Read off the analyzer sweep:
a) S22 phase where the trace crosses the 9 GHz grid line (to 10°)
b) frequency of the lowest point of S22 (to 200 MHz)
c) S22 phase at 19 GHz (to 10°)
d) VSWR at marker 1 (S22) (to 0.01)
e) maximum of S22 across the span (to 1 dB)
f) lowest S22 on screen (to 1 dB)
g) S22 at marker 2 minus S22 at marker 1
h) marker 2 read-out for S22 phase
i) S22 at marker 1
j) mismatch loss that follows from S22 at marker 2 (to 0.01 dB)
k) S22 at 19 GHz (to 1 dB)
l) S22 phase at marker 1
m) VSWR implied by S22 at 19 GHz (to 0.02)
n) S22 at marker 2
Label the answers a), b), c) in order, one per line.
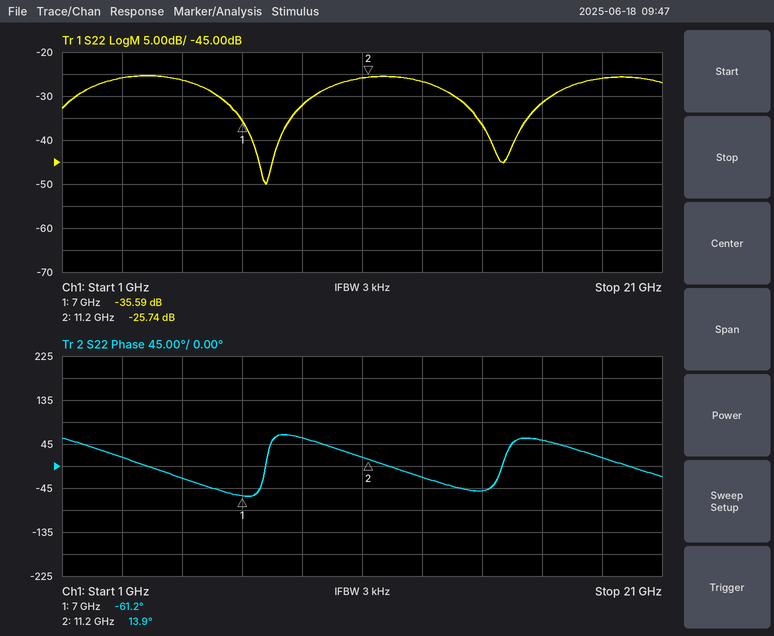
a) 60°
b) 7.8 GHz
c) 20°
d) 1.03
e) -25 dB
f) -50 dB
g) 9.85 dB
h) 13.9°
i) -35.59 dB
j) 0.01 dB
k) -26 dB
l) -61.2°
m) 1.10
n) -25.74 dB
